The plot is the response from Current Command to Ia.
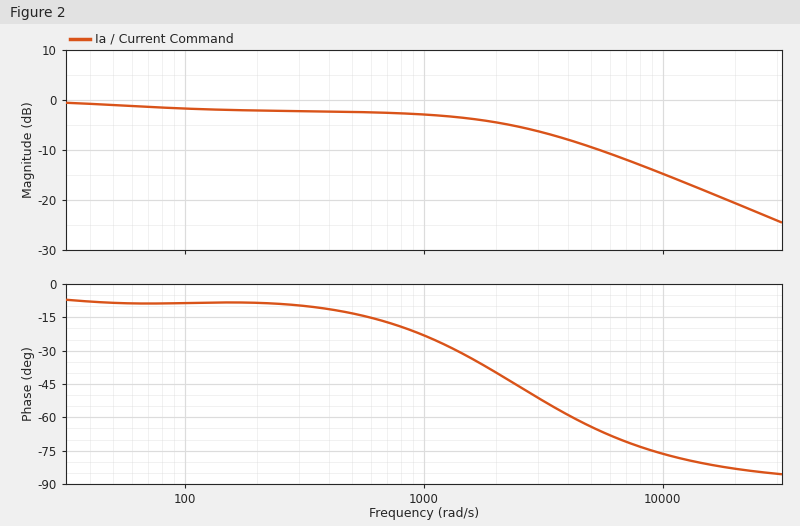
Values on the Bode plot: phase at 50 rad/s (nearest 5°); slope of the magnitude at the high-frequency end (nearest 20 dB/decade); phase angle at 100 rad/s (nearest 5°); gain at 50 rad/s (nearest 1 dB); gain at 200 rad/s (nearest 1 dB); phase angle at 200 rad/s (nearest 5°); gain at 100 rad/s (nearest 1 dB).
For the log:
-10°
-20 dB/decade
-10°
-1 dB
-2 dB
-10°
-2 dB
